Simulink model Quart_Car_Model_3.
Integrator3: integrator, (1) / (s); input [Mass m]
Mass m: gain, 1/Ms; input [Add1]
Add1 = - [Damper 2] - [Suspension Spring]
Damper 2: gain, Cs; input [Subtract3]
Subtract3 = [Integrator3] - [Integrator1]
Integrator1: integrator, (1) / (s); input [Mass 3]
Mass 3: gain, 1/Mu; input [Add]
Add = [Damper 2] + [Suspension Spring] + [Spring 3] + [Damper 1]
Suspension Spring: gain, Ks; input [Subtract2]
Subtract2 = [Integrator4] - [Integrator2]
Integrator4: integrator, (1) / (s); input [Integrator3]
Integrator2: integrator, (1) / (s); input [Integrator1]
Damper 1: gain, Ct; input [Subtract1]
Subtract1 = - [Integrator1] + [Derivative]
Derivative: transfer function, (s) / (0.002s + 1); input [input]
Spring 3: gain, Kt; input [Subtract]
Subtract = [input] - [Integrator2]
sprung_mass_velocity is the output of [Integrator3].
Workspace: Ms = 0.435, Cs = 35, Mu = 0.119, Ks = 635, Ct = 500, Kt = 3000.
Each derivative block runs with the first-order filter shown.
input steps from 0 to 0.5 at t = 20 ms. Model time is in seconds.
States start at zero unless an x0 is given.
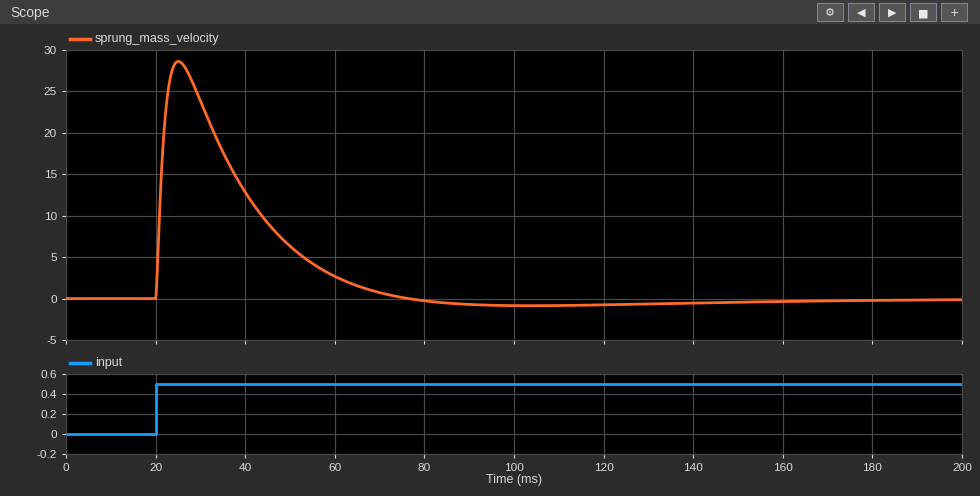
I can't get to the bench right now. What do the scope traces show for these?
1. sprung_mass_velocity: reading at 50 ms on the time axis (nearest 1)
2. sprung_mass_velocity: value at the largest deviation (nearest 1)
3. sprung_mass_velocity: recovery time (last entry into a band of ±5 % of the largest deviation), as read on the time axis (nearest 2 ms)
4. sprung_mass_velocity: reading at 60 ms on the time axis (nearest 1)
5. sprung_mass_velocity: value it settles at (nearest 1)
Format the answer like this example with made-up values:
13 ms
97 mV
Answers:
6
29
66 ms
3
0
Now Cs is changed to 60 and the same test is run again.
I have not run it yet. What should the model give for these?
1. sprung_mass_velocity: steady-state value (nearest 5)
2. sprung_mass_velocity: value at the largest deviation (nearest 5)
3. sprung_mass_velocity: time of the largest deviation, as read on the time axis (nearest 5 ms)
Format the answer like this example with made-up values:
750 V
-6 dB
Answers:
0
40
25 ms
